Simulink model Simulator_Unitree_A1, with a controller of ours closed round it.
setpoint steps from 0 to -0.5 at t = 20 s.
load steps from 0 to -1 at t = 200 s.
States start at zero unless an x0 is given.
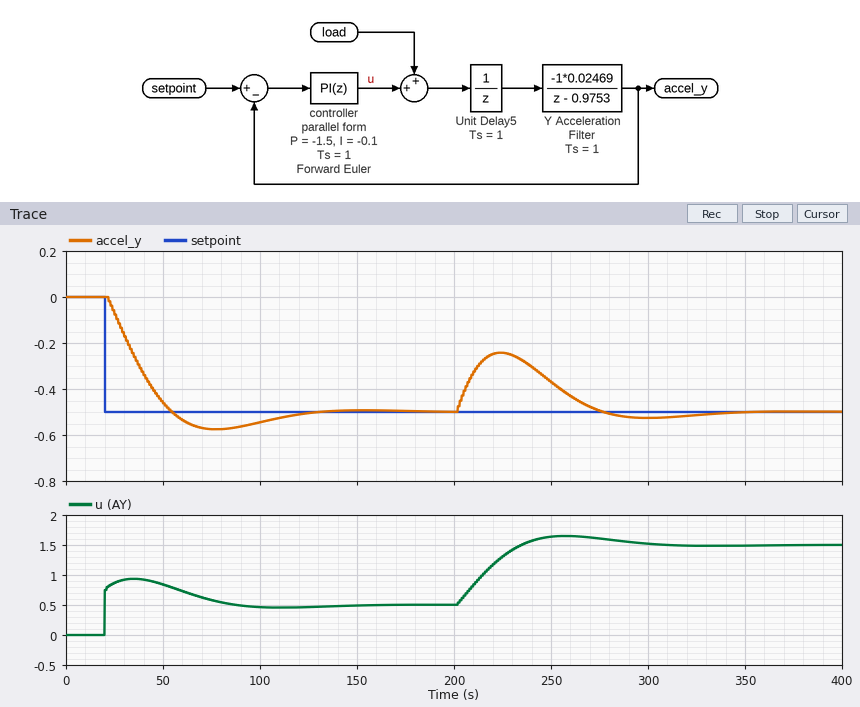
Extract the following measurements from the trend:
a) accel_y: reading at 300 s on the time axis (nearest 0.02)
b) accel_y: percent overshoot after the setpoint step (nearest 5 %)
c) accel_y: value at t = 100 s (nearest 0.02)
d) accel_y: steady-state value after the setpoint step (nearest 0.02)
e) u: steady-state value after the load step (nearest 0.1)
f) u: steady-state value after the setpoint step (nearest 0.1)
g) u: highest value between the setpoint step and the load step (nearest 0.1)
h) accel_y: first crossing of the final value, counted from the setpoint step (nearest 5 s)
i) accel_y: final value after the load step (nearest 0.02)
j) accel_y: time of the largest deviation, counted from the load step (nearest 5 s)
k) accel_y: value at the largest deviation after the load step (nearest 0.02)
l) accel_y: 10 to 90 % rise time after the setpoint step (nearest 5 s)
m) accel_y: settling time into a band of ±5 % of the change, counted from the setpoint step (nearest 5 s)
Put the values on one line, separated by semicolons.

-0.52; 15 %; -0.54; -0.50; 1.5; 0.5; 0.9; 35 s; -0.50; 25 s; -0.24; 25 s; 90 s
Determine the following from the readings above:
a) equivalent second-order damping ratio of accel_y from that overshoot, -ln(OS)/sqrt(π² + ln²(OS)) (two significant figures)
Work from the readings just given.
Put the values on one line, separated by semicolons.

0.52
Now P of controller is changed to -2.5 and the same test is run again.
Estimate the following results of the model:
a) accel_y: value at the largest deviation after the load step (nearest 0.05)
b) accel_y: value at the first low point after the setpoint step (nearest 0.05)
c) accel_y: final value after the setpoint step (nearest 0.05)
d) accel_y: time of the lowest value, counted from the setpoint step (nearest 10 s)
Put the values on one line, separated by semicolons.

-0.30; -0.55; -0.50; 50 s
